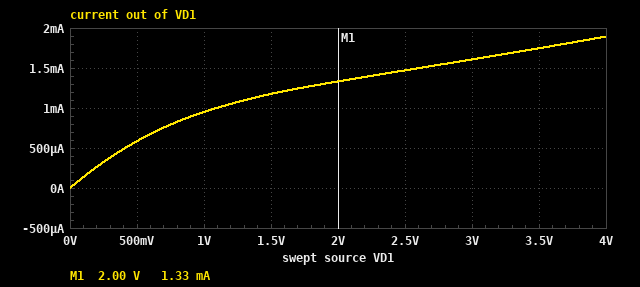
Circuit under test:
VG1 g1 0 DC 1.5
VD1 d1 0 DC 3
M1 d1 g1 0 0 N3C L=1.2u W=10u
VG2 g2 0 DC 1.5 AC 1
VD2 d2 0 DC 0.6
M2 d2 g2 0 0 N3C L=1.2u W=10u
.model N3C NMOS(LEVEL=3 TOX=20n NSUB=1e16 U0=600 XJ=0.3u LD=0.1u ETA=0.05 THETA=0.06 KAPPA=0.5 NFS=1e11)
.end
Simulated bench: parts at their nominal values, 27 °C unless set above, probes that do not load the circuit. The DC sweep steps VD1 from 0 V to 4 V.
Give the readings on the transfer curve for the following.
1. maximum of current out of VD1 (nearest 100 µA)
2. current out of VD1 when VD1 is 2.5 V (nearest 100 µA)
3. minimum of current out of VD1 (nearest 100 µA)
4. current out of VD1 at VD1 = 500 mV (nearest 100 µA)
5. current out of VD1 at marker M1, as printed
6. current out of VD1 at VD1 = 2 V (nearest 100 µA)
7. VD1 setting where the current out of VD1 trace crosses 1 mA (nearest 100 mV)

1.9 mA
1.5 mA
0 A
600 µA
1.33 mA
1.3 mA
1.1 V
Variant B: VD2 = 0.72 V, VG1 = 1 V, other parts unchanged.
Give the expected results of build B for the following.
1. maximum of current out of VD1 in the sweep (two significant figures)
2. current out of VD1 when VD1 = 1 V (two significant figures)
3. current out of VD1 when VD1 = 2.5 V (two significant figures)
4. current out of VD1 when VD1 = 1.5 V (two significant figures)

960 µA
520 µA
740 µA
600 µA
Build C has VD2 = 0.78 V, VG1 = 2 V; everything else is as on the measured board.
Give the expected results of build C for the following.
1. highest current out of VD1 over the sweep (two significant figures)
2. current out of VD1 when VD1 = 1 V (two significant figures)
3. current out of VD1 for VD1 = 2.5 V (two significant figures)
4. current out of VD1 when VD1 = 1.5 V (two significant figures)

3.0 mA
1.4 mA
2.3 mA
1.8 mA
